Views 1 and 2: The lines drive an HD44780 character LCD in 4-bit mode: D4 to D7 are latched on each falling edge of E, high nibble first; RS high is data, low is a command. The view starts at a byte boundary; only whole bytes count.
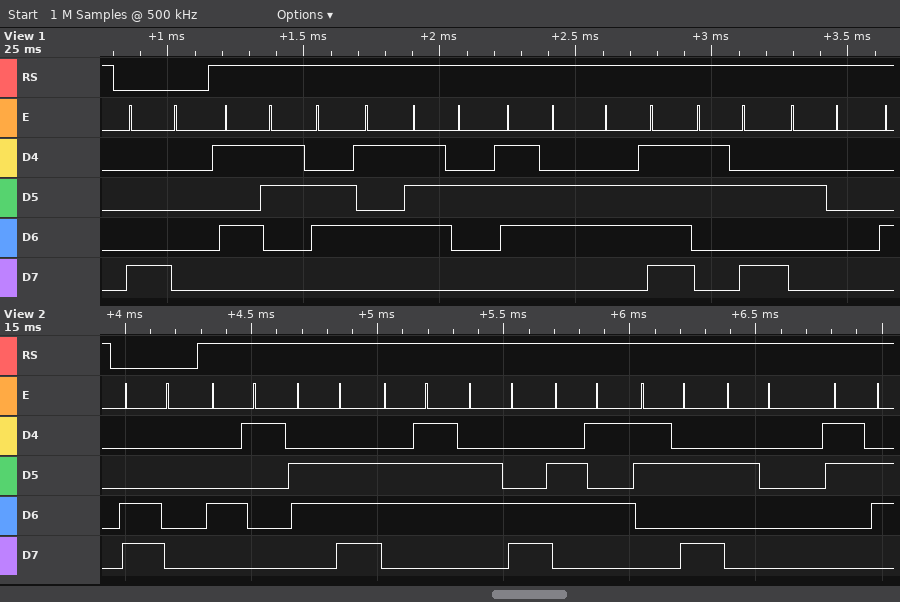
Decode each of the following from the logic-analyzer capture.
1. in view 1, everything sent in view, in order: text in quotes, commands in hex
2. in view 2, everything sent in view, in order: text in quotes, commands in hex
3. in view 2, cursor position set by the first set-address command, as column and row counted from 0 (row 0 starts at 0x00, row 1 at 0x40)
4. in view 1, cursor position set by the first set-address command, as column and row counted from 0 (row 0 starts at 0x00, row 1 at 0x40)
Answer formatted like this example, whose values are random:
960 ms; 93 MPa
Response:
0x80 "Servo: "; 0xC0 "Angle: 6"; column 0, row 1; column 0, row 0
